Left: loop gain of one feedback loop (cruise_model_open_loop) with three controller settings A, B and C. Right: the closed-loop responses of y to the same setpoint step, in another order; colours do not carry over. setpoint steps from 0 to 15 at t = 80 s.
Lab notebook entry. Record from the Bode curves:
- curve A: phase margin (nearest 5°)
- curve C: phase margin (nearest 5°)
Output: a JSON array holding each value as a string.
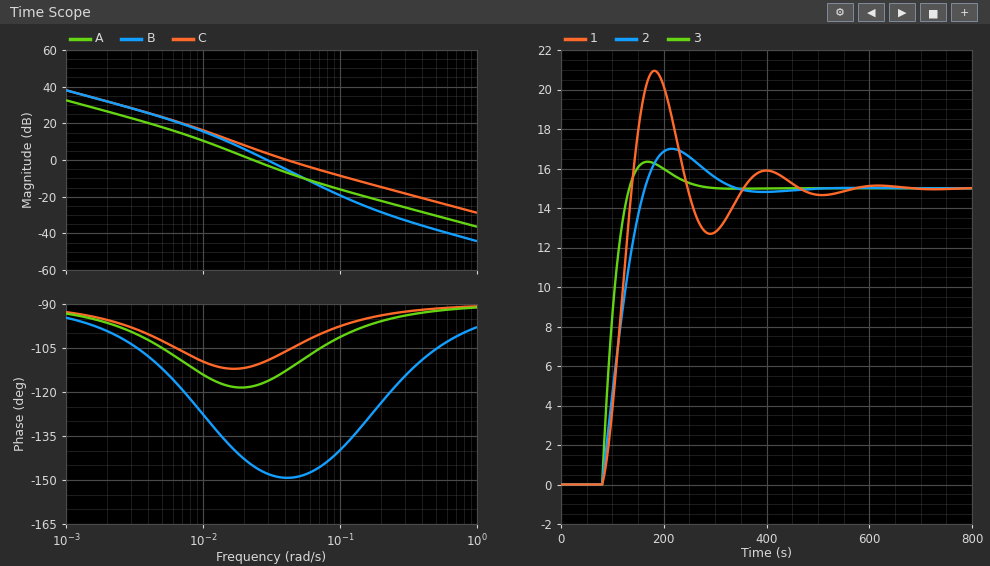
["60°", "75°"]
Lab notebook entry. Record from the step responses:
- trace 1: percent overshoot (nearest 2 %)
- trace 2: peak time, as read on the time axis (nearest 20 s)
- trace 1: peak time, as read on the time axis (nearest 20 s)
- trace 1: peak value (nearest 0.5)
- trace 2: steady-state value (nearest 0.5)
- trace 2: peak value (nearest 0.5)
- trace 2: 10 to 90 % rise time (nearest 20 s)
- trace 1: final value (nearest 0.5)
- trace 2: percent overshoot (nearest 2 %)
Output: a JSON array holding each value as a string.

["40 %", "220 s", "180 s", "21.0", "15.0", "17.0", "60 s", "15.0", "14 %"]
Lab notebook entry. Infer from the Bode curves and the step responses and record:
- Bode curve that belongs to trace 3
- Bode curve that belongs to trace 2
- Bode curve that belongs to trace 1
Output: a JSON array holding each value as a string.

["C", "A", "B"]
